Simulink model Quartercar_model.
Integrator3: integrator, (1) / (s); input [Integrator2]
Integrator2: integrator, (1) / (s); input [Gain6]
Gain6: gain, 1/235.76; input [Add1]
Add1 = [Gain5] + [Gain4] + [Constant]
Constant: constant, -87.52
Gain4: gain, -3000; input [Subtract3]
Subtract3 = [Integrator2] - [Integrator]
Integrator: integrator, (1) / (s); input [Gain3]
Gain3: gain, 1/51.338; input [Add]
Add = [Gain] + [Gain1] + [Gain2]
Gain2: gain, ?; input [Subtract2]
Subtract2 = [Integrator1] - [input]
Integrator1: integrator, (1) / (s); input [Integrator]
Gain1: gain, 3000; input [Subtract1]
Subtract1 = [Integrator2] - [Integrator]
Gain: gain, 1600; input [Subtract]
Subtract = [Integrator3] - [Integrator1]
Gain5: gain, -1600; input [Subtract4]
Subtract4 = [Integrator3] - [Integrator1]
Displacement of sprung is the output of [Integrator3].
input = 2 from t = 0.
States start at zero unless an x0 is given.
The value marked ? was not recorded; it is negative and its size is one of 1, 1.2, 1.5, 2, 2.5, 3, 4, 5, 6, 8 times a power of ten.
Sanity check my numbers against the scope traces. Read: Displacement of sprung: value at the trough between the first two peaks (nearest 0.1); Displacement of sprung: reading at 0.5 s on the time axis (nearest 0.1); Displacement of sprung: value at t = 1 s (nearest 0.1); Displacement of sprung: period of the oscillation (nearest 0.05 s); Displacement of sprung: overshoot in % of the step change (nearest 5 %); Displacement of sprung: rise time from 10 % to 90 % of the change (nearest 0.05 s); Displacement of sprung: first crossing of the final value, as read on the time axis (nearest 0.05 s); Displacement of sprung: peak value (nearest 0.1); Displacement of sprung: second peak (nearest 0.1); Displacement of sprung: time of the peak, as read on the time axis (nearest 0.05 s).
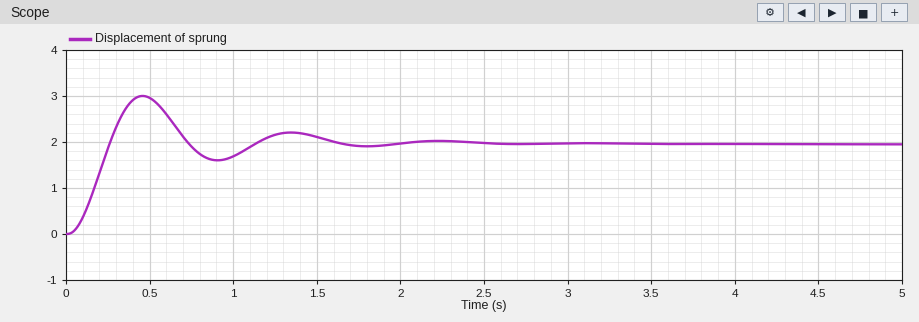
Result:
1.6
3.0
1.7
0.90 s
55 %
0.15 s
0.25 s
3.0
2.2
0.45 s
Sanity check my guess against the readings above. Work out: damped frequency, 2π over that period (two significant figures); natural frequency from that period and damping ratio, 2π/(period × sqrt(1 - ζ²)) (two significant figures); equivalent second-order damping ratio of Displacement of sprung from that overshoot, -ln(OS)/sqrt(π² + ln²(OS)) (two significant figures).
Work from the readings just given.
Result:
7.0 rad/s
7.1 rad/s
0.19
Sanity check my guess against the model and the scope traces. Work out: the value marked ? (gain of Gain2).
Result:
-15000
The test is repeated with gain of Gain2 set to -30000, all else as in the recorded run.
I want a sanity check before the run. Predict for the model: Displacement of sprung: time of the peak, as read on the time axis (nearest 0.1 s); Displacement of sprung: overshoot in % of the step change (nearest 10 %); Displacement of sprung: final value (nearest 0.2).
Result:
0.3 s
40 %
2.0
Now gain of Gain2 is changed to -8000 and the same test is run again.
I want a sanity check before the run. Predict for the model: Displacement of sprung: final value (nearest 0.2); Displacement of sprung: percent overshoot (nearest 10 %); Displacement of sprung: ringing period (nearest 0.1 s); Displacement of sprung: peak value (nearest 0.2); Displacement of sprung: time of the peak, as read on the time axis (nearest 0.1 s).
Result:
2.0
70 %
1.2 s
3.2
0.6 s
